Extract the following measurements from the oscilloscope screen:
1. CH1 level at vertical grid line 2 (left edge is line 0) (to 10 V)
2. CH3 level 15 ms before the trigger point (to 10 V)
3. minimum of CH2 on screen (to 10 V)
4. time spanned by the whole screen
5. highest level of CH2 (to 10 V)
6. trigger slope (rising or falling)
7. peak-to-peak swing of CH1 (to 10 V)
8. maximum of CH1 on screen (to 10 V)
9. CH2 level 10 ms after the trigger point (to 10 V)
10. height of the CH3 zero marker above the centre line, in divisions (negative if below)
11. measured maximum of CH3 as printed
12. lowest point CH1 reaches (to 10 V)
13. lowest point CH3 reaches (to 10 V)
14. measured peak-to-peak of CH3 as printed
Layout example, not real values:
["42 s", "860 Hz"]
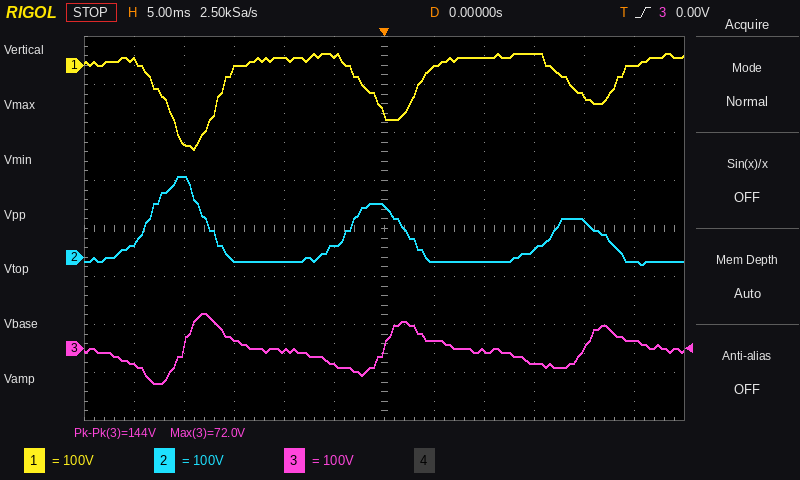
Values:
["-160 V", "20 V", "-20 V", "60 ms", "170 V", "rising", "200 V", "20 V", "-10 V", "-2.5 div", "72.0 V", "-180 V", "-70 V", "144 V"]
